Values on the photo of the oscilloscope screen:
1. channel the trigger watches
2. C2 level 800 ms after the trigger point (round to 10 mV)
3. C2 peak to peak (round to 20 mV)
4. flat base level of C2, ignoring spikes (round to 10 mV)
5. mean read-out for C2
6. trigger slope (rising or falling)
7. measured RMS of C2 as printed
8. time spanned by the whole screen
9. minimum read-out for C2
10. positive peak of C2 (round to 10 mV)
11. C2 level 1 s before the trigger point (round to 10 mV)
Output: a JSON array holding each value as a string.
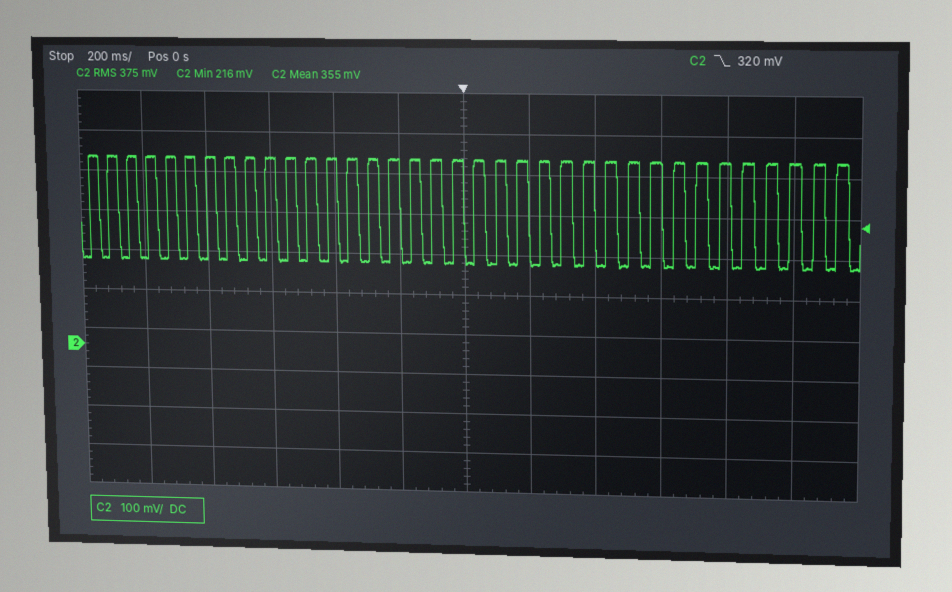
["C2", "480 mV", "260 mV", "220 mV", "355 mV", "falling", "375 mV", "2.4 s", "216 mV", "480 mV", "220 mV"]
